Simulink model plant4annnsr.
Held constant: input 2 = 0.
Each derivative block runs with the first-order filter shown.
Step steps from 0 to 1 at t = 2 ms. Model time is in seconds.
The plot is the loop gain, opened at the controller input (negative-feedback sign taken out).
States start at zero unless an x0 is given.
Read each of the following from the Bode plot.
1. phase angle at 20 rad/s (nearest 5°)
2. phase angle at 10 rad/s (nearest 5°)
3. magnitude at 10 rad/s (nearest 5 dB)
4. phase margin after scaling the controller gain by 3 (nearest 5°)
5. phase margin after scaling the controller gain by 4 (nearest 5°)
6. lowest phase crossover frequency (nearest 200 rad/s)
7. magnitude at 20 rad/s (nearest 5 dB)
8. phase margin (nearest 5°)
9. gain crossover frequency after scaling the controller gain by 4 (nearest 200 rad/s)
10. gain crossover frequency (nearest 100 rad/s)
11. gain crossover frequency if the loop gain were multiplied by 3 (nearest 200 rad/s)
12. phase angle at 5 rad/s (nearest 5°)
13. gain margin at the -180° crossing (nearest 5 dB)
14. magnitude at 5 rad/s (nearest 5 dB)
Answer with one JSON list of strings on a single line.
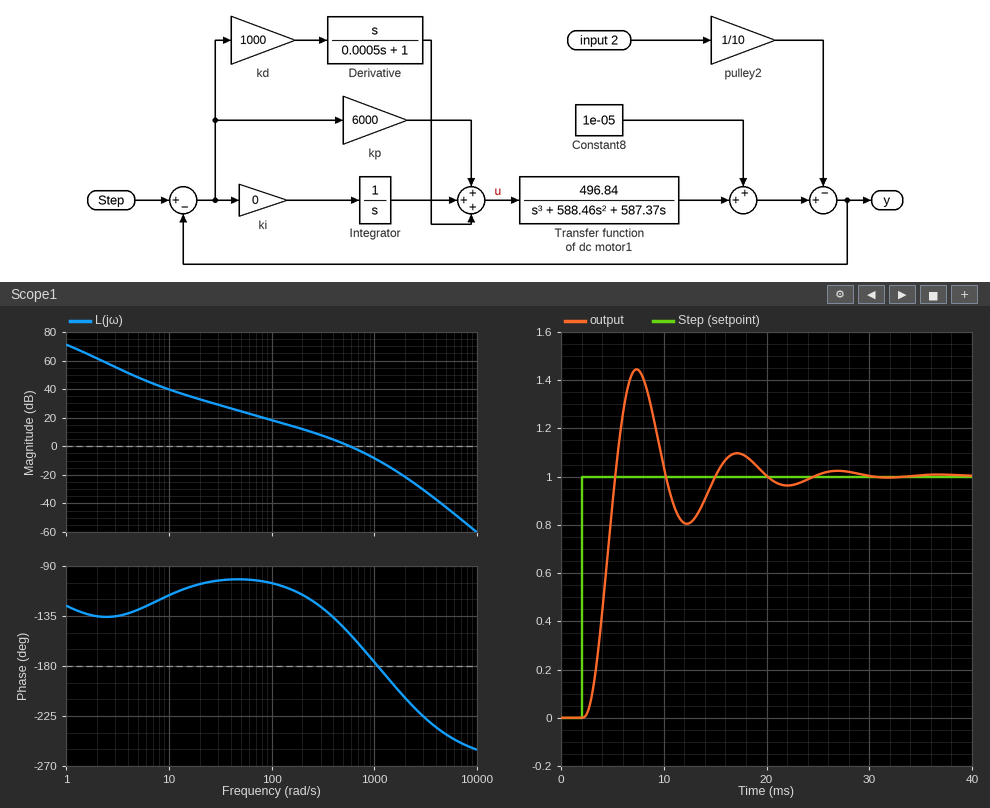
["-105°", "-115°", "40 dB", "0°", "-5°", "1000 rad/s", "35 dB", "30°", "1200 rad/s", "600 rad/s", "1000 rad/s", "-130°", "10 dB", "50 dB"]
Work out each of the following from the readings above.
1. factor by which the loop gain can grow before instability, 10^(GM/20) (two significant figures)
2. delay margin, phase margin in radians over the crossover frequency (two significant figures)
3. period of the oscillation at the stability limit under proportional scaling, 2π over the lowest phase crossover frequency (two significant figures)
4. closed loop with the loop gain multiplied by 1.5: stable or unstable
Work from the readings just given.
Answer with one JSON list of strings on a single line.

["3.2", "0.00087 s", "0.0063 s", "stable"]
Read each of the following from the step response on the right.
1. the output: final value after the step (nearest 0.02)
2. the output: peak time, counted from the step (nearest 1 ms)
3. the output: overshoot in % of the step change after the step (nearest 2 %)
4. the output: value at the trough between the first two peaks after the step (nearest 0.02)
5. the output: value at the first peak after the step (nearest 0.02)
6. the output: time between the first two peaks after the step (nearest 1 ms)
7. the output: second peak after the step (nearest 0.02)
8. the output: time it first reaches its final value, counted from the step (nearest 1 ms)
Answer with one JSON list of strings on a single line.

["1.00", "5 ms", "44 %", "0.80", "1.44", "10 ms", "1.10", "3 ms"]
